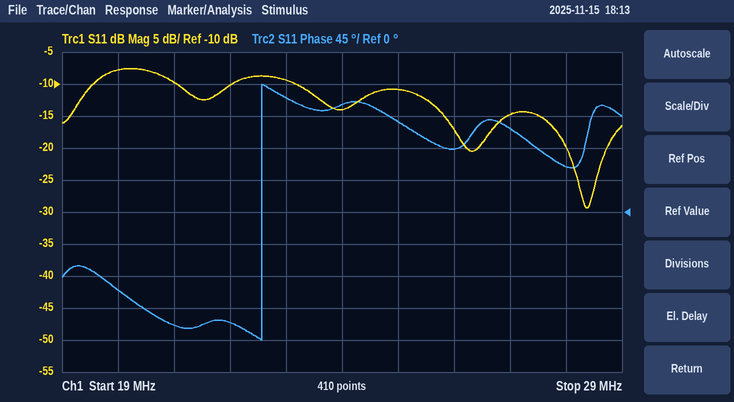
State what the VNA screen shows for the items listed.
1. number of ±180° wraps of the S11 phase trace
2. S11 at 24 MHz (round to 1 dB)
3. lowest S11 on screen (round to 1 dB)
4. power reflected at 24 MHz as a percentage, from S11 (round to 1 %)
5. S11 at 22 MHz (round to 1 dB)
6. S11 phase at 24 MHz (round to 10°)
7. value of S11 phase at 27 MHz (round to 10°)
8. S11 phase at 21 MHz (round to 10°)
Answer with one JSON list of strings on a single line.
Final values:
["1", "-14 dB", "-29 dB", "4 %", "-10 dB", "150°", "120°", "-160°"]
